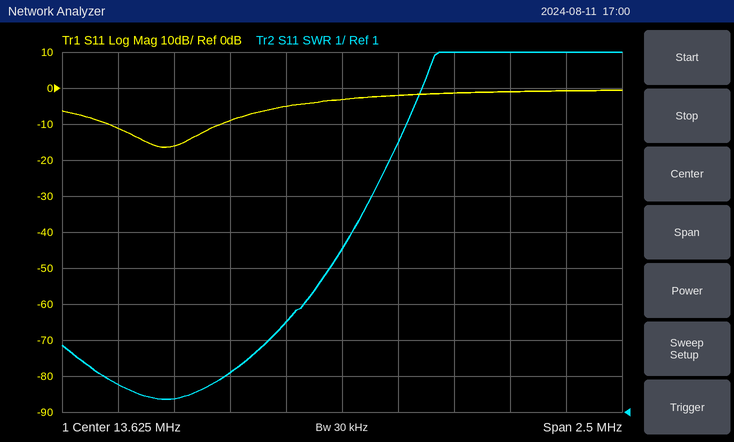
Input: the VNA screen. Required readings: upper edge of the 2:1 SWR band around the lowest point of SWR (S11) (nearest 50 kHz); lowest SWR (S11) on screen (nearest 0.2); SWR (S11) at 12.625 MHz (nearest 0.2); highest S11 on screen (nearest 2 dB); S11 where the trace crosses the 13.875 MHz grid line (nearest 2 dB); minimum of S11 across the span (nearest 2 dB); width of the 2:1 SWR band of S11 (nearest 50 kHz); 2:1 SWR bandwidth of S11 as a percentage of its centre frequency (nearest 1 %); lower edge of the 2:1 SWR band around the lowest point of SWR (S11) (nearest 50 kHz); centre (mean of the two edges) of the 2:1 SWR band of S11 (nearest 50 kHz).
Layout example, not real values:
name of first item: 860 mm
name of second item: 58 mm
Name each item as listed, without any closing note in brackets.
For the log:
upper edge of the 2:1 SWR band around the lowest point of SWR (S11): 13.10 MHz
lowest SWR (S11) on screen: 1.4
SWR (S11) at 12.625 MHz: 1.8
highest S11 on screen: 0 dB
S11 where the trace crosses the 13.875 MHz grid line: -2 dB
minimum of S11 across the span: -16 dB
width of the 2:1 SWR band of S11: 550 kHz
2:1 SWR bandwidth of S11 as a percentage of its centre frequency: 4 %
lower edge of the 2:1 SWR band around the lowest point of SWR (S11): 12.55 MHz
centre (mean of the two edges) of the 2:1 SWR band of S11: 12.85 MHz
